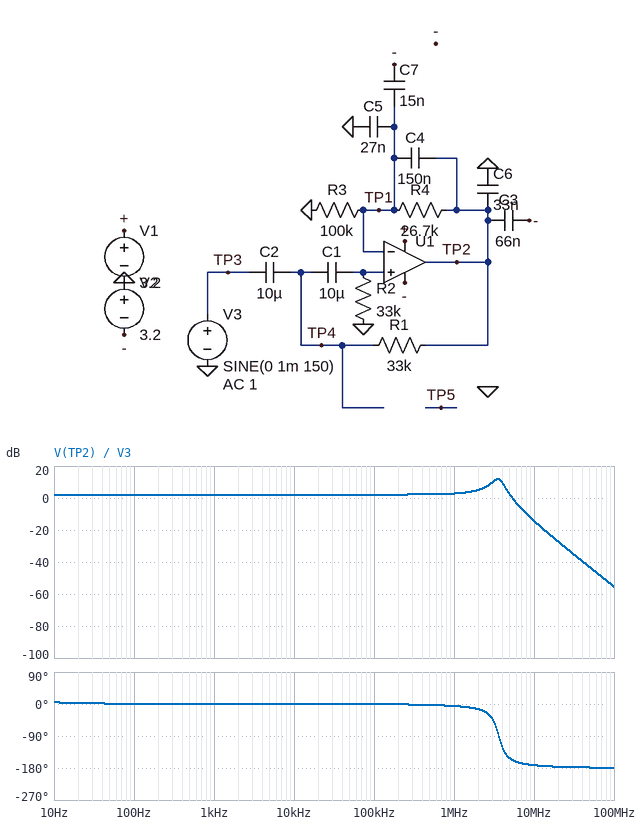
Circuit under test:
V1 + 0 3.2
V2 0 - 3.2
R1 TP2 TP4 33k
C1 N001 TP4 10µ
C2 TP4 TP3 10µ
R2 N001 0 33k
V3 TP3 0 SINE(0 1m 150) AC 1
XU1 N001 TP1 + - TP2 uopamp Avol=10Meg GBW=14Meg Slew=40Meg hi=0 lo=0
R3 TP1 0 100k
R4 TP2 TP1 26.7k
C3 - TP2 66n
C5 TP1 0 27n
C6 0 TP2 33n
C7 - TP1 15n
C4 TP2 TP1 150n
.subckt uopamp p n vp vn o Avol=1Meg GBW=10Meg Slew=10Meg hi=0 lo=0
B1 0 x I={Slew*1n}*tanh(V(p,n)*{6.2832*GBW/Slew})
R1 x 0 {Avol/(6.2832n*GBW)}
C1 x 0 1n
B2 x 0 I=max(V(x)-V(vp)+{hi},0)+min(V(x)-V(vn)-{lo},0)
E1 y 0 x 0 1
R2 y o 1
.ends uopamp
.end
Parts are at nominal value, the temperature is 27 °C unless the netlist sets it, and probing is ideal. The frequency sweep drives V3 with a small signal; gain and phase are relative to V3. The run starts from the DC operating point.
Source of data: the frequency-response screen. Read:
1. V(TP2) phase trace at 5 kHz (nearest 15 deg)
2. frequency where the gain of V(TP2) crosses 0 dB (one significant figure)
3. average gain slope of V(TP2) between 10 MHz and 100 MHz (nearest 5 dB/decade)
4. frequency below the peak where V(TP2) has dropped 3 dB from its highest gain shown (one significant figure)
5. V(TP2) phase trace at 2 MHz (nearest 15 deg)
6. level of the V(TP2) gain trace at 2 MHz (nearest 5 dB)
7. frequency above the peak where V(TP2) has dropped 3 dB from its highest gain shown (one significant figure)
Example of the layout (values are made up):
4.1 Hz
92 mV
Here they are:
0 deg
5 MHz
-40 dB/decade
3 MHz
-15 deg
5 dB
4 MHz
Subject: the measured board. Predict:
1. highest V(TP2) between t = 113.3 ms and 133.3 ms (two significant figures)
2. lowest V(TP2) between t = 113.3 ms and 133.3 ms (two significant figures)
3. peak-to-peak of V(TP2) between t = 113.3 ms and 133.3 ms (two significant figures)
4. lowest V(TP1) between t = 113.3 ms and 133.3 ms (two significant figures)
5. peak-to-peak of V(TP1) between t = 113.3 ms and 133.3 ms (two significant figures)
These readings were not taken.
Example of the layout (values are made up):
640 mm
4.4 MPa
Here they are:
1.3 mV
-1.3 mV
2.6 mV
-1.0 mV
2.0 mV
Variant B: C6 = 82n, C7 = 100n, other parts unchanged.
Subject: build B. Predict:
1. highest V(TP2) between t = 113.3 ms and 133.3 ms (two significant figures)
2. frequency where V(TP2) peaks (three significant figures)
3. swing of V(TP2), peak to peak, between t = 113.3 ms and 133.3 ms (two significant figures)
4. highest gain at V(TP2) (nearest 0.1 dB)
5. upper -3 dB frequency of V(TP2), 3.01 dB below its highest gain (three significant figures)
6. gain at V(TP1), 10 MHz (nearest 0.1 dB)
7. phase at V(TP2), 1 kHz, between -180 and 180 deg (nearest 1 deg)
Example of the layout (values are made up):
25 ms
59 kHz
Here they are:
1.8 mV
2.30 MHz
3.6 mV
15.6 dB
2.65 MHz
-24.6 dB
1 deg
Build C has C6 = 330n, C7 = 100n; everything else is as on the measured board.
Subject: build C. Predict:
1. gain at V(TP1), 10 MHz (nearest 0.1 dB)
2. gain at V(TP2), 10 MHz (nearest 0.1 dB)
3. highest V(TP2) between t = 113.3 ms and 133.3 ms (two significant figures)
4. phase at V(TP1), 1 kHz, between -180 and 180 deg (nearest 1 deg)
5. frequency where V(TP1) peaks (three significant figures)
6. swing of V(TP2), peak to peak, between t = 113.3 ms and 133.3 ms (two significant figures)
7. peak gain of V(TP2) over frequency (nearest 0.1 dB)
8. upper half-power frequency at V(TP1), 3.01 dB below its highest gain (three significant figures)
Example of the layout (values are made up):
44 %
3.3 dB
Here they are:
-31.5 dB
-26.2 dB
1.8 mV
0 deg
1.59 MHz
3.6 mV
18.8 dB
1.76 MHz
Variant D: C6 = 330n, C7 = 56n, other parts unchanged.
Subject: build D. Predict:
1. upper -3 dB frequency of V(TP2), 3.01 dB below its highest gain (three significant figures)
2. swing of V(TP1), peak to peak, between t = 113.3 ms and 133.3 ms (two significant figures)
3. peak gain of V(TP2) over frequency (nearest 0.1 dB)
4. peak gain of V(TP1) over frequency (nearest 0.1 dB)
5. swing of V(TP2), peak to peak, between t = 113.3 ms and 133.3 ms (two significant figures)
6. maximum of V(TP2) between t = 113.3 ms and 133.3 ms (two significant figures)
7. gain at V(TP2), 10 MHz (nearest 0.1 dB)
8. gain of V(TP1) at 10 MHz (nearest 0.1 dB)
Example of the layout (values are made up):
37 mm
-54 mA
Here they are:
1.94 MHz
2.0 mV
17.9 dB
14.1 dB
3.1 mV
1.5 mV
-25.8 dB
-29.6 dB
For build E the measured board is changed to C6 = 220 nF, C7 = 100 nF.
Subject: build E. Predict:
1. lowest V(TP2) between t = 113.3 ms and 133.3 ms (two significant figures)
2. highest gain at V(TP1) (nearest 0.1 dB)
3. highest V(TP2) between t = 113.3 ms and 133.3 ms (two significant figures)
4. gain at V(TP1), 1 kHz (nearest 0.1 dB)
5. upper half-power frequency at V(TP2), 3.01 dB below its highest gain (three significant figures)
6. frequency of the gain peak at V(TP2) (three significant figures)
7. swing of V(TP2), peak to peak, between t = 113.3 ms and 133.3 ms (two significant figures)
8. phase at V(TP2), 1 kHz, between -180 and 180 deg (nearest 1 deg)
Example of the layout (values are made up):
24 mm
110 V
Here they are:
-1.8 mV
12.3 dB
1.8 mV
0 dB
2.03 MHz
1.82 MHz
3.6 mV
1 deg
